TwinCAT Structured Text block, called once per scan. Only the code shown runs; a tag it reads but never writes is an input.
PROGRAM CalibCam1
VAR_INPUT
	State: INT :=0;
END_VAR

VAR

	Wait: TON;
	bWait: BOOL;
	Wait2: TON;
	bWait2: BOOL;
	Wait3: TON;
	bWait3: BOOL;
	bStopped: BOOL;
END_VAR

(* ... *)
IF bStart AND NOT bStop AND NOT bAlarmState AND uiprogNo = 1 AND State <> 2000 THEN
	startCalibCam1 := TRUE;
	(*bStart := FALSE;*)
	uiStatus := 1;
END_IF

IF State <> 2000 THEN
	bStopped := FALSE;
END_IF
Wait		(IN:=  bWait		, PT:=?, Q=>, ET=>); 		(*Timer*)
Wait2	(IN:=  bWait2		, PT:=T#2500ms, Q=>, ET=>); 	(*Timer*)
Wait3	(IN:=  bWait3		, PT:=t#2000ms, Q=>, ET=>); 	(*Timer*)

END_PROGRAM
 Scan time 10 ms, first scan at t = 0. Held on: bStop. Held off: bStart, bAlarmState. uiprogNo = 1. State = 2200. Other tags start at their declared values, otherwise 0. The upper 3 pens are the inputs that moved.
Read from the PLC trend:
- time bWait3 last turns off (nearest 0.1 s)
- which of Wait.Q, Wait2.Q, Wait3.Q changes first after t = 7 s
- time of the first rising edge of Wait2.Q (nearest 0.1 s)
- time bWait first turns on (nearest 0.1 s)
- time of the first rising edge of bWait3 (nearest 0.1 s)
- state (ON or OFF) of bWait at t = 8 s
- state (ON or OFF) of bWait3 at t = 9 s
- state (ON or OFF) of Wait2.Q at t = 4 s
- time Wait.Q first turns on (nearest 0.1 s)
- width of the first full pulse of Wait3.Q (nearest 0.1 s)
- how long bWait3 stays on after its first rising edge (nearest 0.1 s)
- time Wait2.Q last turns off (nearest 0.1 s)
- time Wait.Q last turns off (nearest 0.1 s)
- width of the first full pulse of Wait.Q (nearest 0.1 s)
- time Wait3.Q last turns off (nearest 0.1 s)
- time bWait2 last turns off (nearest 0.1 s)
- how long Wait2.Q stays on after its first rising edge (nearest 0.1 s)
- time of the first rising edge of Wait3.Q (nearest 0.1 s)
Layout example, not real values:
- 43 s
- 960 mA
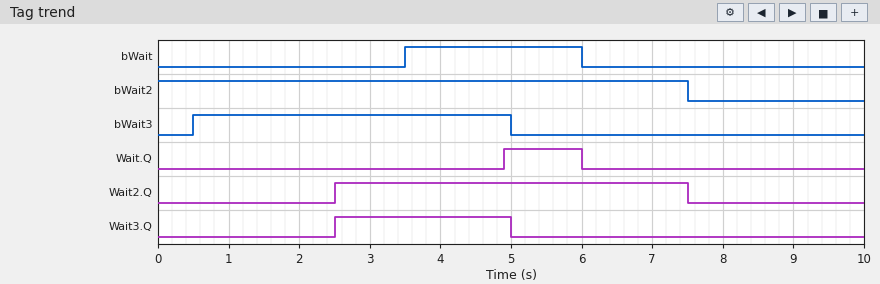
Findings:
- 5.0 s
- Wait2.Q
- 2.5 s
- 3.5 s
- 0.5 s
- OFF
- OFF
- ON
- 4.9 s
- 2.5 s
- 4.5 s
- 7.5 s
- 6.0 s
- 1.1 s
- 5.0 s
- 7.5 s
- 5.0 s
- 2.5 s
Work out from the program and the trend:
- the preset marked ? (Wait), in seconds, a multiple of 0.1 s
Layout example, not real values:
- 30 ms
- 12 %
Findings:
- 1.4 s
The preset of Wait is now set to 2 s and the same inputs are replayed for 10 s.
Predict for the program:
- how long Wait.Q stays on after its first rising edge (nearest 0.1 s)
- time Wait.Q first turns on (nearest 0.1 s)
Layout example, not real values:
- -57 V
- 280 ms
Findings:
- 0.5 s
- 5.5 s
